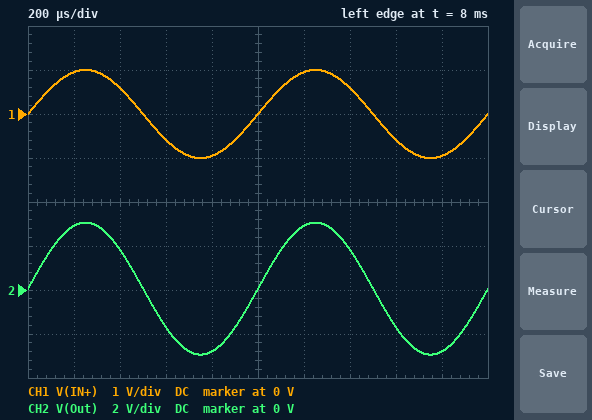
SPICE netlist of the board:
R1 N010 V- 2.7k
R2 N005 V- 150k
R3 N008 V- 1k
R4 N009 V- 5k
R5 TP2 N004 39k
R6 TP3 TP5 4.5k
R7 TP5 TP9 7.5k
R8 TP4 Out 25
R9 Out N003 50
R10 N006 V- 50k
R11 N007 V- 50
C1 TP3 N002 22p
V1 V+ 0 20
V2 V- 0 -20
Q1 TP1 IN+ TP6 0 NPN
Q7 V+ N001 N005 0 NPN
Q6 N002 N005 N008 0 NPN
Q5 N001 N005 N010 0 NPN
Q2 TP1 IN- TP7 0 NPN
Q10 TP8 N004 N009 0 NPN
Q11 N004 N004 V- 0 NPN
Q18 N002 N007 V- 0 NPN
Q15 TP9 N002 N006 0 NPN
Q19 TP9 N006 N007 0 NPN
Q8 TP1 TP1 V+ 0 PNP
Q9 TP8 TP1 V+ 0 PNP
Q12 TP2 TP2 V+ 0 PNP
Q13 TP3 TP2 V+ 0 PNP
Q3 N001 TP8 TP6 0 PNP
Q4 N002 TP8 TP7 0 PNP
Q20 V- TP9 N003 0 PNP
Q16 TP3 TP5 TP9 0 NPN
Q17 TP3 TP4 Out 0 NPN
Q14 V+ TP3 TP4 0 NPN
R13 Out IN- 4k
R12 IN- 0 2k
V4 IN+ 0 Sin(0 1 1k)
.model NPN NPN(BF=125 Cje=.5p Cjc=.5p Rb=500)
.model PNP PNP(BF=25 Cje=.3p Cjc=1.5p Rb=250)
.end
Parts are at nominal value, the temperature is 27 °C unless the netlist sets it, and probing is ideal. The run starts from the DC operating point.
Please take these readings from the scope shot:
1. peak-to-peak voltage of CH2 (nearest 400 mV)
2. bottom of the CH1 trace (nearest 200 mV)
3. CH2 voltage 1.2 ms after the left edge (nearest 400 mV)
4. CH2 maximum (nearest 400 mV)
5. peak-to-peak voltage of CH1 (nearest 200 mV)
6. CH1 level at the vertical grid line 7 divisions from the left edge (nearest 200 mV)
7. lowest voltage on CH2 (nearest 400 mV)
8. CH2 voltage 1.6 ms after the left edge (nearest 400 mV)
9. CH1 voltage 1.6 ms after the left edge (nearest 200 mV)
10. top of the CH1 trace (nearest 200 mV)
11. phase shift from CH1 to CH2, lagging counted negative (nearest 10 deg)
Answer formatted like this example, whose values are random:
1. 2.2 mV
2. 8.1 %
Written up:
1. 6.0 V
2. -1.0 V
3. 2.8 V
4. 3.2 V
5. 2.0 V
6. 600 mV
7. -2.8 V
8. -1.6 V
9. -600 mV
10. 1.0 V
11. 0 deg
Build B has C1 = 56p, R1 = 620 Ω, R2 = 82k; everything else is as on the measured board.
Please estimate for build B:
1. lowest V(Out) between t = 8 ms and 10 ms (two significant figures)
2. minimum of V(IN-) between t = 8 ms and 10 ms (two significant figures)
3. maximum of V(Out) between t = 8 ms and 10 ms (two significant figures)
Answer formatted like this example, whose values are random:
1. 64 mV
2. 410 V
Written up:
1. -3.0 V
2. -1.0 V
3. 3.0 V
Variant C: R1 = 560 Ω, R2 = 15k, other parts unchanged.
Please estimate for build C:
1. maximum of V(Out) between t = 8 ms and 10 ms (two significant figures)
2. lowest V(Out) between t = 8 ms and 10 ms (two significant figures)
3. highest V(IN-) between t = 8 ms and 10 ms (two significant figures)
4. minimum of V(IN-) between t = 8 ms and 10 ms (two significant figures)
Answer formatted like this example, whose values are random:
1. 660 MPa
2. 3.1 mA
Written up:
1. 3.0 V
2. -3.0 V
3. 990 mV
4. -1.0 V
